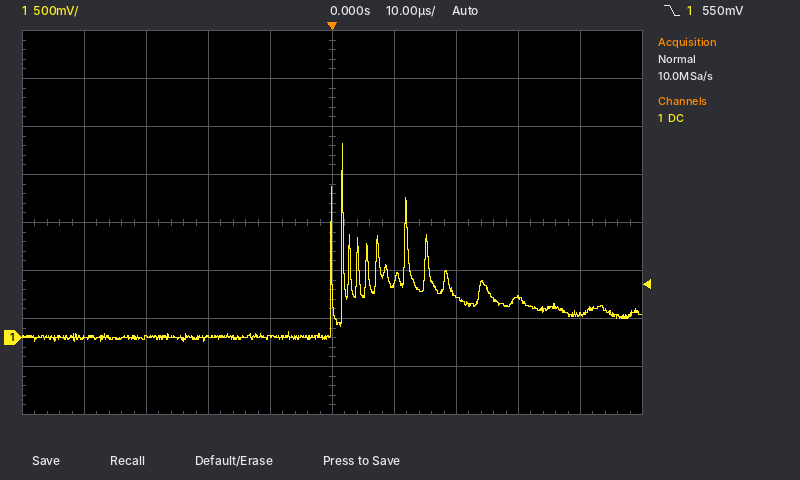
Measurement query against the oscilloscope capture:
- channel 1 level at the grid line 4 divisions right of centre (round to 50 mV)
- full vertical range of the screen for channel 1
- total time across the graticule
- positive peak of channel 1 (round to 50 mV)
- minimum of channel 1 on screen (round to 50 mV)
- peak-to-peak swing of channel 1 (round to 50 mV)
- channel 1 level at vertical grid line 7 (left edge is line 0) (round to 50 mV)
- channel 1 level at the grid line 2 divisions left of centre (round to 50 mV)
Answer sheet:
250 mV
4 V
100 µs
2.00 V
-50 mV
2.05 V
450 mV
0 mV
